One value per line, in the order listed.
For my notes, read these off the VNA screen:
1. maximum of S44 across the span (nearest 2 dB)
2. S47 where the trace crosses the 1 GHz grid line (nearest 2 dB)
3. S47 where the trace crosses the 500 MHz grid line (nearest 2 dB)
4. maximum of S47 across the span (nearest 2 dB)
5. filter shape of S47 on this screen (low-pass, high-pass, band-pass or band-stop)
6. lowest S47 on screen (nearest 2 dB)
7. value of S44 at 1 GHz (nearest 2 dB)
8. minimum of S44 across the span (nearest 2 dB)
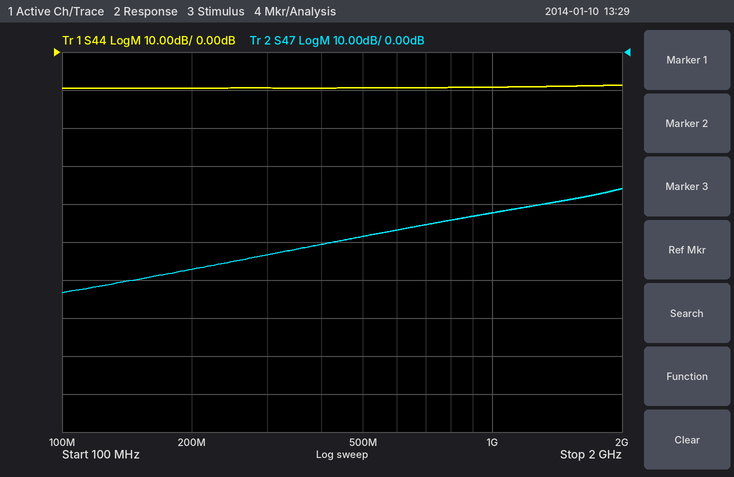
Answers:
-8 dB
-42 dB
-48 dB
-36 dB
high-pass
-64 dB
-10 dB
-10 dB
